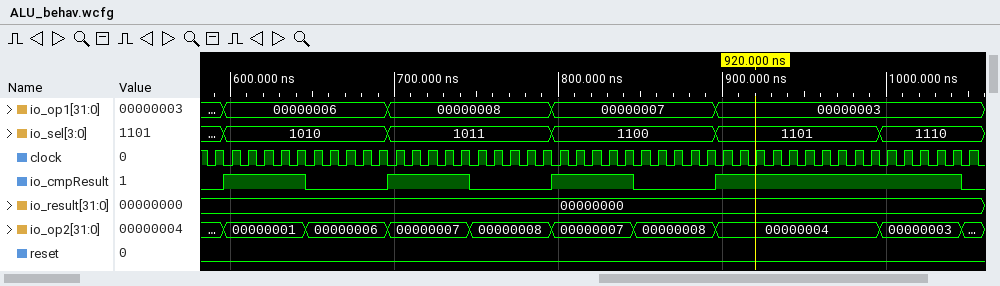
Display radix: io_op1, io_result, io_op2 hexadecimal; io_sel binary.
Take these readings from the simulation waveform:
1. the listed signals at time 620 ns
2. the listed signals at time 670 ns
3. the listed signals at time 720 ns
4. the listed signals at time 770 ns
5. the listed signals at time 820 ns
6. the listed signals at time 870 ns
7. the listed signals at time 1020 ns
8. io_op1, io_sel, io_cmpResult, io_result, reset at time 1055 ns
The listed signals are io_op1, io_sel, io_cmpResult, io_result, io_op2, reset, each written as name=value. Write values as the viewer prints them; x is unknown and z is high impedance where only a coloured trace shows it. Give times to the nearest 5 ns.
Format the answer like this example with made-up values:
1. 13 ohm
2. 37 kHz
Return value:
1. io_op1=00000006, io_sel=1010, io_cmpResult=1, io_result=00000000, io_op2=00000001, reset=0
2. io_op1=00000006, io_sel=1010, io_cmpResult=0, io_result=00000000, io_op2=00000006, reset=0
3. io_op1=00000008, io_sel=1011, io_cmpResult=1, io_result=00000000, io_op2=00000007, reset=0
4. io_op1=00000008, io_sel=1011, io_cmpResult=0, io_result=00000000, io_op2=00000008, reset=0
5. io_op1=00000007, io_sel=1100, io_cmpResult=1, io_result=00000000, io_op2=00000007, reset=0
6. io_op1=00000007, io_sel=1100, io_cmpResult=0, io_result=00000000, io_op2=00000008, reset=0
7. io_op1=00000003, io_sel=1110, io_cmpResult=1, io_result=00000000, io_op2=00000003, reset=0
8. io_op1=00000003, io_sel=1110, io_cmpResult=0, io_result=00000000, reset=0
